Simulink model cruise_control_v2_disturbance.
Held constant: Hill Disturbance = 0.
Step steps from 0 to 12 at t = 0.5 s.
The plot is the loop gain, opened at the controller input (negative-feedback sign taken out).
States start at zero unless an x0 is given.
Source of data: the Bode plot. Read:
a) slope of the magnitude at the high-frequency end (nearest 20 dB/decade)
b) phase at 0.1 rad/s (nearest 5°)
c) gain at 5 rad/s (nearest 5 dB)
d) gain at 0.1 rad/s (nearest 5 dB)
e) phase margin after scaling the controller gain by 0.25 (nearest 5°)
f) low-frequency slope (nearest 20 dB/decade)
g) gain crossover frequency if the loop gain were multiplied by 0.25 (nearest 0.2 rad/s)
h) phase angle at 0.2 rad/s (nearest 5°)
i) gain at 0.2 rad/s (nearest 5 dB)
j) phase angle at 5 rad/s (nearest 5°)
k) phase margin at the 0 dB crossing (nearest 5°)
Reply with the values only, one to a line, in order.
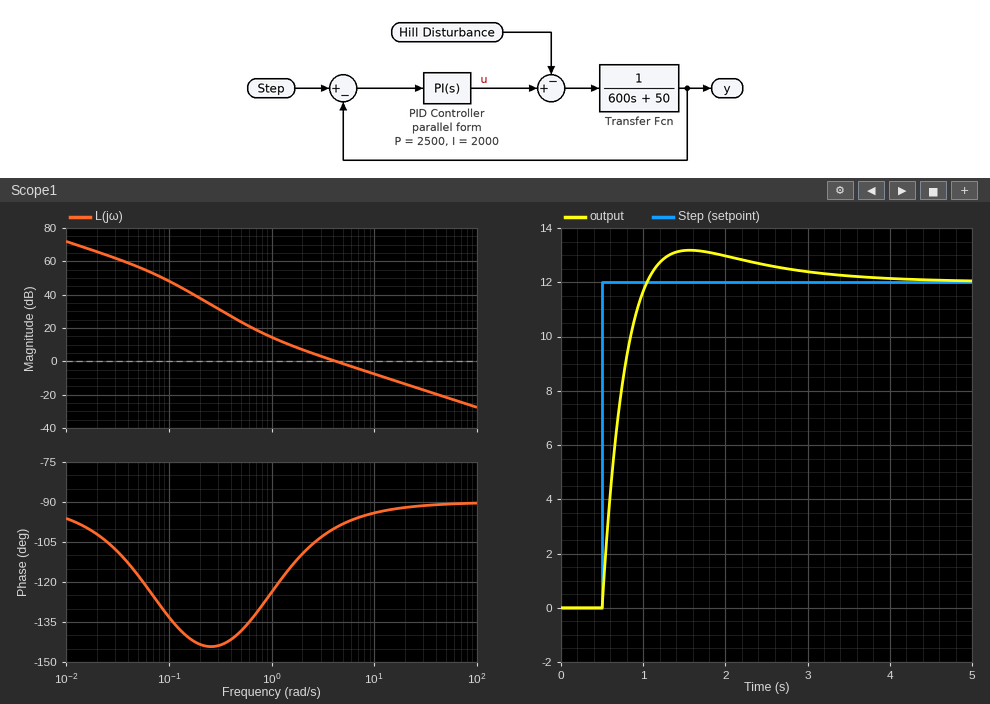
-20 dB/decade
-135°
0 dB
50 dB
60°
-20 dB/decade
1.2 rad/s
-145°
40 dB
-100°
80°
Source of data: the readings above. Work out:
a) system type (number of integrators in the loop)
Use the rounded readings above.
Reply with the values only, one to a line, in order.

1
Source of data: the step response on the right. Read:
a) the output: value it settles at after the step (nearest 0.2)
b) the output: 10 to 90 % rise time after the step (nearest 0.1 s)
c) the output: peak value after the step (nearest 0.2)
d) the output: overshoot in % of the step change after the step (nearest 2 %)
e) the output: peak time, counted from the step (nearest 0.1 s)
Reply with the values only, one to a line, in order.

12.0
0.4 s
13.2
10 %
1.1 s
